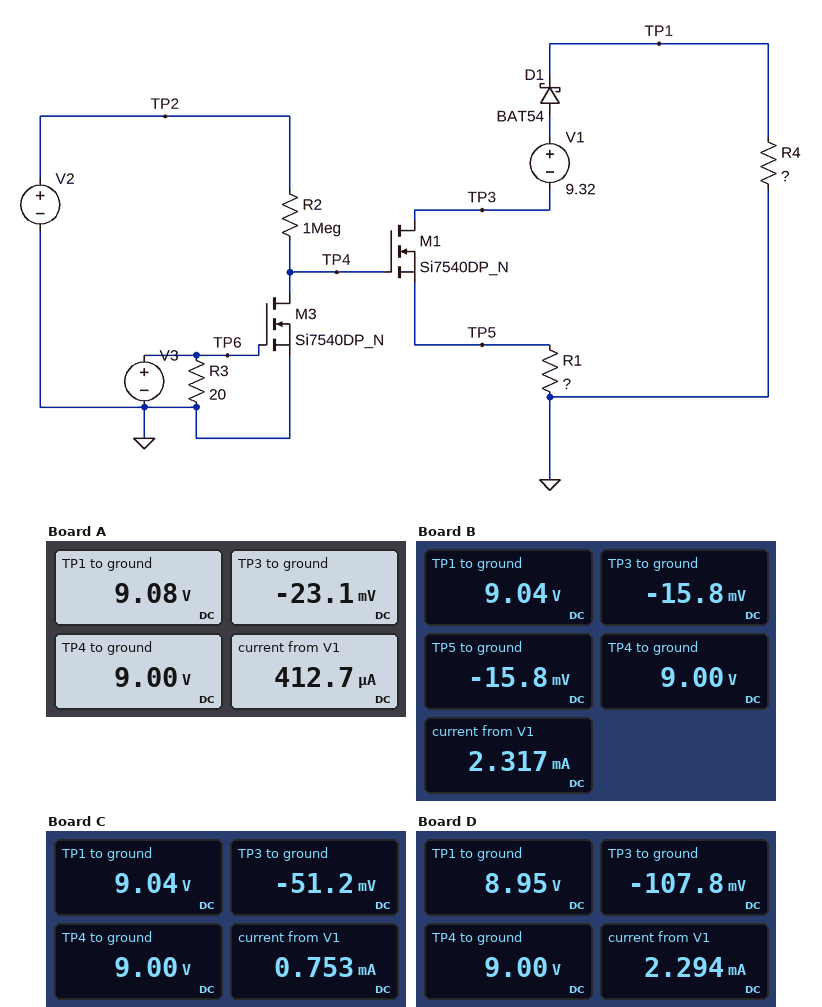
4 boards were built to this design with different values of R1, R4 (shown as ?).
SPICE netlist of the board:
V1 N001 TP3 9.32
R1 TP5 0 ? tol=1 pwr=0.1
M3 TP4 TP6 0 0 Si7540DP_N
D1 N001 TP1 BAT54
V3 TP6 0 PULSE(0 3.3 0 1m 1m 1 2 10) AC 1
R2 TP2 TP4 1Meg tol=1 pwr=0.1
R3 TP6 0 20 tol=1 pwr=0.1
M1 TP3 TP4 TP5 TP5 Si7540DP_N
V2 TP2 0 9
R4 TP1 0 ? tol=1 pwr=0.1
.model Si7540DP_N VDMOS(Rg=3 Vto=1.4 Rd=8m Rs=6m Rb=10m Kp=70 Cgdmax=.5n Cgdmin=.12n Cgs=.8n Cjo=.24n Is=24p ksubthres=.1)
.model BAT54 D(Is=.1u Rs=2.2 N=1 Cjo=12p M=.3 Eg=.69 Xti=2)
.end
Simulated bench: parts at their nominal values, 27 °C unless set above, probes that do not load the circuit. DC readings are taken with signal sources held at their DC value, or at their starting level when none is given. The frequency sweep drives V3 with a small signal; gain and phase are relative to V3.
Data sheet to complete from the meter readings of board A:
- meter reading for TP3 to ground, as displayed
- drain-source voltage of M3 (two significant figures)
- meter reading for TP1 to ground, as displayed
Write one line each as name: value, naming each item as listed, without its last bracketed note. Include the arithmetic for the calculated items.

meter reading for TP3 to ground, as displayed: -23.1 mV
drain-source voltage of M3: 9 V = 9.0 V
meter reading for TP1 to ground, as displayed: 9.08 V
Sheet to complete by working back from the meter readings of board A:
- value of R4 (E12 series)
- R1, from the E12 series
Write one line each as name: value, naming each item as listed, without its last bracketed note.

value of R4: 22 kΩ
R1, from the E12 series: 56 Ω
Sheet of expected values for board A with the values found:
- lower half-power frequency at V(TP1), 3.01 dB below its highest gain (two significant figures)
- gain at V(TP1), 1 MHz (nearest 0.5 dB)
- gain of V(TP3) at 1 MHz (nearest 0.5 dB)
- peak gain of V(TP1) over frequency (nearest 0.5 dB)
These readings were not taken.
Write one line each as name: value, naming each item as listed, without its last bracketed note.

lower half-power frequency at V(TP1), 3.01 dB below its highest gain: 11 MHz
gain at V(TP1), 1 MHz: -27.5 dB
gain of V(TP3) at 1 MHz: -27.5 dB
peak gain of V(TP1) over frequency: -6.0 dB
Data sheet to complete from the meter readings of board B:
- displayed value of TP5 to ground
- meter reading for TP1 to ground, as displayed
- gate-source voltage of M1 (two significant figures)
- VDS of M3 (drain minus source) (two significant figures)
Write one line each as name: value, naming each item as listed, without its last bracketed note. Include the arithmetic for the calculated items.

displayed value of TP5 to ground: -15.8 mV
meter reading for TP1 to ground, as displayed: 9.04 V
gate-source voltage of M1: 9 V - (-15.8 mV) = 9.0 V
VDS of M3 (drain minus source): 9 V = 9.0 V
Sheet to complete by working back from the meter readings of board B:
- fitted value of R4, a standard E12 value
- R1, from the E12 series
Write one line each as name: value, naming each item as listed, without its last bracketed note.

fitted value of R4, a standard E12 value: 3.9 kΩ
R1, from the E12 series: 6.8 Ω
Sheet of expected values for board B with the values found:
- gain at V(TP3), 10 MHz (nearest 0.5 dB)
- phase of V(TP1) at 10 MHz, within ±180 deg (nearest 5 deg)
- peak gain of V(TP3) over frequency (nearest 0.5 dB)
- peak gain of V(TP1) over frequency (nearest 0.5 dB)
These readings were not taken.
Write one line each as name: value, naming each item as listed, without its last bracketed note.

gain at V(TP3), 10 MHz: -26.0 dB
phase of V(TP1) at 10 MHz, within ±180 deg: 75 deg
peak gain of V(TP3) over frequency: -15.0 dB
peak gain of V(TP1) over frequency: -15.0 dB
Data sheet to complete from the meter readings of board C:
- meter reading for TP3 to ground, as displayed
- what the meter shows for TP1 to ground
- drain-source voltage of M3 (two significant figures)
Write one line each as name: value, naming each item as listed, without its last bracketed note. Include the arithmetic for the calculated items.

meter reading for TP3 to ground, as displayed: -51.2 mV
what the meter shows for TP1 to ground: 9.04 V
drain-source voltage of M3: 9 V = 9.0 V
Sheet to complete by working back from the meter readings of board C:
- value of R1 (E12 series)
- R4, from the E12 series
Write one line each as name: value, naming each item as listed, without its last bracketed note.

value of R1: 68 Ω
R4, from the E12 series: 12 kΩ
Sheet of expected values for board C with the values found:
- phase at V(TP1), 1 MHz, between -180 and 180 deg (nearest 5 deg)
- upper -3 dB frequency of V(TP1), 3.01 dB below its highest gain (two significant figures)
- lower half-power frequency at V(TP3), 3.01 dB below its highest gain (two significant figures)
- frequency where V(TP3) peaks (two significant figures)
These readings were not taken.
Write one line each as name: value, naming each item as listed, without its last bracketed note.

phase at V(TP1), 1 MHz, between -180 and 180 deg: 85 deg
upper -3 dB frequency of V(TP1), 3.01 dB below its highest gain: 86 MHz
lower half-power frequency at V(TP3), 3.01 dB below its highest gain: 9.3 MHz
frequency where V(TP3) peaks: 28 MHz
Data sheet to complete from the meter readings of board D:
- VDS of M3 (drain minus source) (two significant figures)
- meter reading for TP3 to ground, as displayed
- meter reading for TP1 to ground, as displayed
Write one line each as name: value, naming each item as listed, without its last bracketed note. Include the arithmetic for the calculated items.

VDS of M3 (drain minus source): 9 V = 9.0 V
meter reading for TP3 to ground, as displayed: -107.8 mV
meter reading for TP1 to ground, as displayed: 8.95 V
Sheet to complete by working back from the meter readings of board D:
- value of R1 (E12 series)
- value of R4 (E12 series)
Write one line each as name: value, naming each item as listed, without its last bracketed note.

value of R1: 47 Ω
value of R4: 3.9 kΩ
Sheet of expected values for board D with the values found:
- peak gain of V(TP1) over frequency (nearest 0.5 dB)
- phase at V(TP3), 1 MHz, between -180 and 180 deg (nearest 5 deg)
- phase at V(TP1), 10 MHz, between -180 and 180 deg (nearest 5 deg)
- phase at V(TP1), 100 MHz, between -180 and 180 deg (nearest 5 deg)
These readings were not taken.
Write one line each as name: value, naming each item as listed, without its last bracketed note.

peak gain of V(TP1) over frequency: -6.5 dB
phase at V(TP3), 1 MHz, between -180 and 180 deg: 85 deg
phase at V(TP1), 10 MHz, between -180 and 180 deg: 50 deg
phase at V(TP1), 100 MHz, between -180 and 180 deg: -45 deg
